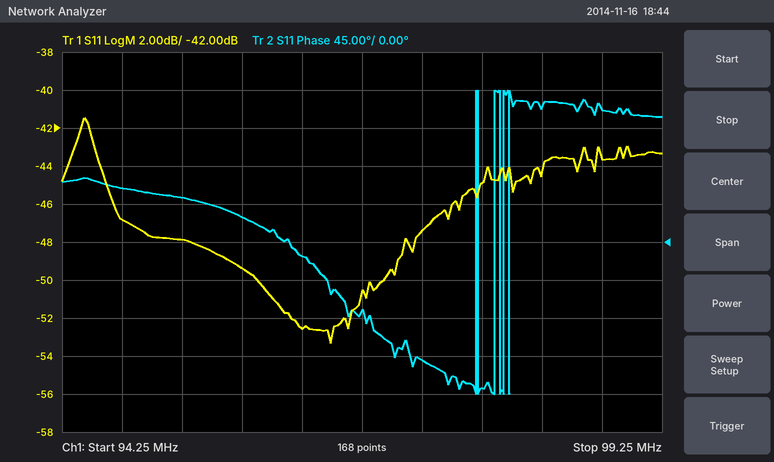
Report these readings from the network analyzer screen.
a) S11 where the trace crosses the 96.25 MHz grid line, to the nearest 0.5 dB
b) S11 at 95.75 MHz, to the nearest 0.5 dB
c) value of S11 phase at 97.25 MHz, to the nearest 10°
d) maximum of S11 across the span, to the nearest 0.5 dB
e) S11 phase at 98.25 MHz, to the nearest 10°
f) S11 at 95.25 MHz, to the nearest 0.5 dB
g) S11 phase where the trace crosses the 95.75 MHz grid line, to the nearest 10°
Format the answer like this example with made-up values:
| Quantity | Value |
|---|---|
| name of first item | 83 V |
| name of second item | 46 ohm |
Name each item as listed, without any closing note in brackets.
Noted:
| Quantity | Value |
|---|---|
| S11 where the trace crosses the 96.25 MHz grid line, to the nearest 0.5 dB | -52.5 dB |
| S11 at 95.75 MHz, to the nearest 0.5 dB | -49.5 dB |
| value of S11 phase at 97.25 MHz, to the nearest 10° | -140° |
| maximum of S11 across the span, to the nearest 0.5 dB | -41.5 dB |
| S11 phase at 98.25 MHz, to the nearest 10° | 160° |
| S11 at 95.25 MHz, to the nearest 0.5 dB | -48.0 dB |
| S11 phase where the trace crosses the 95.75 MHz grid line, to the nearest 10° | 30° |
